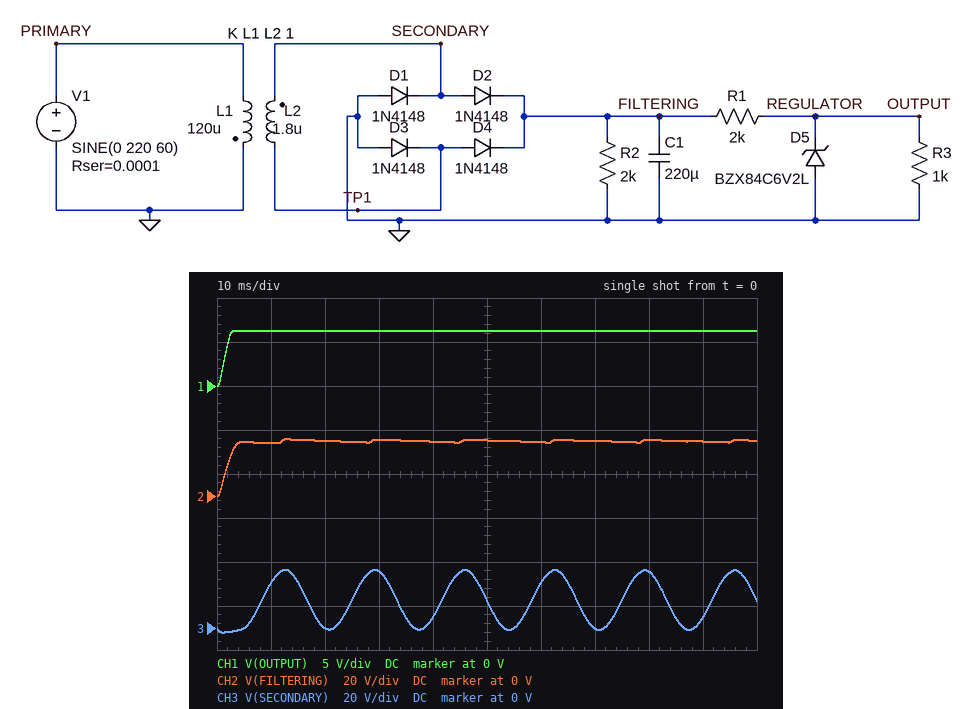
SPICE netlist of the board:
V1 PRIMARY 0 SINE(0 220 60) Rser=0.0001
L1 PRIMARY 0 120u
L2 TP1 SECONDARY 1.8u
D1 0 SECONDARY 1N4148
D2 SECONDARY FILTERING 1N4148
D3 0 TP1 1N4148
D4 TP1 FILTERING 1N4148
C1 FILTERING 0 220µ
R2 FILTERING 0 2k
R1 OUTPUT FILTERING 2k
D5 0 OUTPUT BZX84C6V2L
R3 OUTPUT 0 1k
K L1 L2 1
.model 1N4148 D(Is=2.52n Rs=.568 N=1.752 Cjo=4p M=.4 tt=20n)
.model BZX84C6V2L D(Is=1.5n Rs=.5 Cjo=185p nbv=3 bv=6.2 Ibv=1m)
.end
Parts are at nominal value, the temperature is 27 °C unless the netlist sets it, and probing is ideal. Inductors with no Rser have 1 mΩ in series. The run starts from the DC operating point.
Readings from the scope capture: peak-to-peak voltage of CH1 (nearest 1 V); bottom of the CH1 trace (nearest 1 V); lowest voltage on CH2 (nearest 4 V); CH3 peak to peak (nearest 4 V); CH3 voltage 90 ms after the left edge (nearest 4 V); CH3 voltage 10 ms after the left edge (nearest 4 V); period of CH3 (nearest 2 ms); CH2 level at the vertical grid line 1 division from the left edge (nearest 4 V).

6 V
0 V
0 V
28 V
4 V
20 V
16 ms
24 V
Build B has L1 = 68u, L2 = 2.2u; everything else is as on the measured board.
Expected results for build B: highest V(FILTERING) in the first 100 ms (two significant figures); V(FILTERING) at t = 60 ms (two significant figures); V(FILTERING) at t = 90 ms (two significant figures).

39 V
36 V
37 V
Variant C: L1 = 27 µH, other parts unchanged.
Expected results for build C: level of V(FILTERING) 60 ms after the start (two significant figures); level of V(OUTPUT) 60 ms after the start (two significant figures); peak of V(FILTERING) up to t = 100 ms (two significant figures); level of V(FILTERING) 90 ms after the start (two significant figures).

53 V
6.4 V
58 V
54 V
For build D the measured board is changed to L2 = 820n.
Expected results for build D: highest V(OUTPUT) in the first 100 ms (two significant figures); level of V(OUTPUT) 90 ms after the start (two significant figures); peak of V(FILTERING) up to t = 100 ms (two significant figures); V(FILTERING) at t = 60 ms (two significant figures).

5.6 V
5.4 V
17 V
16 V
